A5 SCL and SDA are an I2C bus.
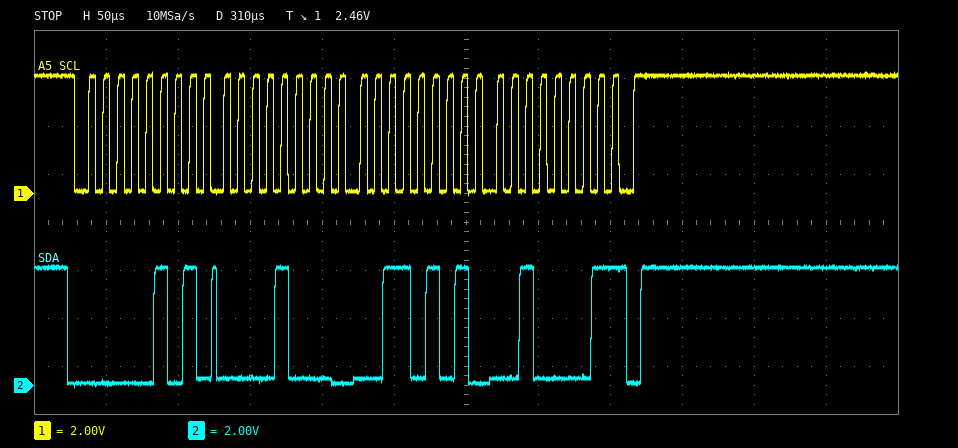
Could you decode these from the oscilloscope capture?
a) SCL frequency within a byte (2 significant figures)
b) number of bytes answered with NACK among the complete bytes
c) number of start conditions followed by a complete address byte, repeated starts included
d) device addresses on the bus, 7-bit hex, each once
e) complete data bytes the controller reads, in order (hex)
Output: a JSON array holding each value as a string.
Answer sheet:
["100 kHz", "1", "1", "0x02", "08 35 21"]
